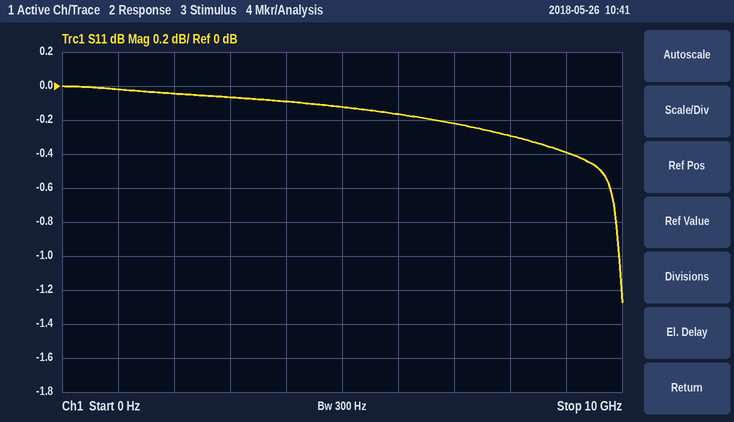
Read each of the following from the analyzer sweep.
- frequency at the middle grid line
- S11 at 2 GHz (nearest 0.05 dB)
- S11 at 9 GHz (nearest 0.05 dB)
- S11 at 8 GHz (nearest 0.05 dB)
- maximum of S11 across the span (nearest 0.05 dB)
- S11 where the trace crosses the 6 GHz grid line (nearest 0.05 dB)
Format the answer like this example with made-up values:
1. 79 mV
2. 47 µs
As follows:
1. 5 GHz
2. -0.05 dB
3. -0.40 dB
4. -0.30 dB
5. 0.00 dB
6. -0.15 dB
